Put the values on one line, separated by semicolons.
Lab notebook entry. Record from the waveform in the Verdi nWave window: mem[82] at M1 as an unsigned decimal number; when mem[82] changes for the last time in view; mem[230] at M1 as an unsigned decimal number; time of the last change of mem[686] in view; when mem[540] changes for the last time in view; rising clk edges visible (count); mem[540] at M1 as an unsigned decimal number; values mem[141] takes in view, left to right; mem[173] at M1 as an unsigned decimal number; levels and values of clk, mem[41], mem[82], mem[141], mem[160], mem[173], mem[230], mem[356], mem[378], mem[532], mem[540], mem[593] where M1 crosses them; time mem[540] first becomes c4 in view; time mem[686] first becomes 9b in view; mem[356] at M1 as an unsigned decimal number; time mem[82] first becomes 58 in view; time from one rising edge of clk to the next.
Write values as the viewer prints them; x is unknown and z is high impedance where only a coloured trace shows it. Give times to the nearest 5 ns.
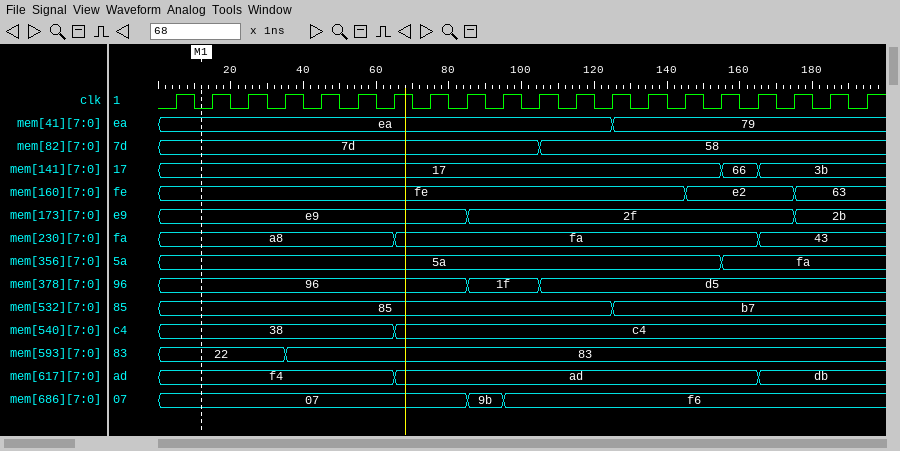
125; 105 ns; 168; 95 ns; 65 ns; 20; 56; 17, 66, 3b; 233; clk=0, mem[41]=ea, mem[82]=7d, mem[141]=17, mem[160]=fe, mem[173]=e9, mem[230]=a8, mem[356]=5a, mem[378]=96, mem[532]=85, mem[540]=38, mem[593]=22; 65 ns; 85 ns; 90; 105 ns; 10 ns
